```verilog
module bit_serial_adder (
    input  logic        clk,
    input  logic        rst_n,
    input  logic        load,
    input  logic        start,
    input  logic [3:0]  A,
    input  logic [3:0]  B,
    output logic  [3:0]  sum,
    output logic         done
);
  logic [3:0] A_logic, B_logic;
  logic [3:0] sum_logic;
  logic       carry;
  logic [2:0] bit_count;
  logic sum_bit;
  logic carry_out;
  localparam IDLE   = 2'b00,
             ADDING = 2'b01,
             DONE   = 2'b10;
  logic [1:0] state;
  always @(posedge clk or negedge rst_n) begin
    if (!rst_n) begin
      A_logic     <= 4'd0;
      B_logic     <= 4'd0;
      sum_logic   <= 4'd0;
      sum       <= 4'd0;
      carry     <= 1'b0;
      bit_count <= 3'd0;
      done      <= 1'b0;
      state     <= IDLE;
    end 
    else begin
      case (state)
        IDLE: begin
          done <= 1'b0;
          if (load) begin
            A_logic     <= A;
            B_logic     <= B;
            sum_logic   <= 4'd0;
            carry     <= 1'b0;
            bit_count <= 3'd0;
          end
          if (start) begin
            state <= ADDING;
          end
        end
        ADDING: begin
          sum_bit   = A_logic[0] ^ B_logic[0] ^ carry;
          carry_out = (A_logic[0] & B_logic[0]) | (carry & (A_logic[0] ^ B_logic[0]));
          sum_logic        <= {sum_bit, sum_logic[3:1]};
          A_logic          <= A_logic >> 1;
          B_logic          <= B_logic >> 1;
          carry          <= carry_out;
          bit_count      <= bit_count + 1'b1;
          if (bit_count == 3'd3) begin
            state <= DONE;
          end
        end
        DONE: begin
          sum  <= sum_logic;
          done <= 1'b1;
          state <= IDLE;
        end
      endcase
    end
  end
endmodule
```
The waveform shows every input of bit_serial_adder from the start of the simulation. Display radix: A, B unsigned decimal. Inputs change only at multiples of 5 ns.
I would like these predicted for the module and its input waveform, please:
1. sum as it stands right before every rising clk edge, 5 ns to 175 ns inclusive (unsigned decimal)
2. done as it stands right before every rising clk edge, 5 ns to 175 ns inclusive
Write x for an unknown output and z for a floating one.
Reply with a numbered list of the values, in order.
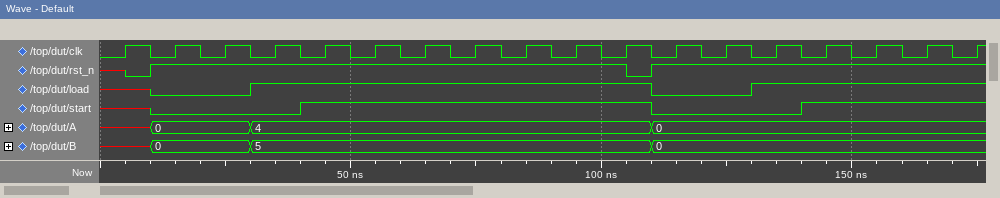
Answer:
1. x, 0, 0, 0, 0, 0, 0, 0, 0, 0, 9, 0, 0, 0, 0, 0, 0, 0
2. x 0 0 0 0 0 0 0 0 0 1 0 0 0 0 0 0 0
